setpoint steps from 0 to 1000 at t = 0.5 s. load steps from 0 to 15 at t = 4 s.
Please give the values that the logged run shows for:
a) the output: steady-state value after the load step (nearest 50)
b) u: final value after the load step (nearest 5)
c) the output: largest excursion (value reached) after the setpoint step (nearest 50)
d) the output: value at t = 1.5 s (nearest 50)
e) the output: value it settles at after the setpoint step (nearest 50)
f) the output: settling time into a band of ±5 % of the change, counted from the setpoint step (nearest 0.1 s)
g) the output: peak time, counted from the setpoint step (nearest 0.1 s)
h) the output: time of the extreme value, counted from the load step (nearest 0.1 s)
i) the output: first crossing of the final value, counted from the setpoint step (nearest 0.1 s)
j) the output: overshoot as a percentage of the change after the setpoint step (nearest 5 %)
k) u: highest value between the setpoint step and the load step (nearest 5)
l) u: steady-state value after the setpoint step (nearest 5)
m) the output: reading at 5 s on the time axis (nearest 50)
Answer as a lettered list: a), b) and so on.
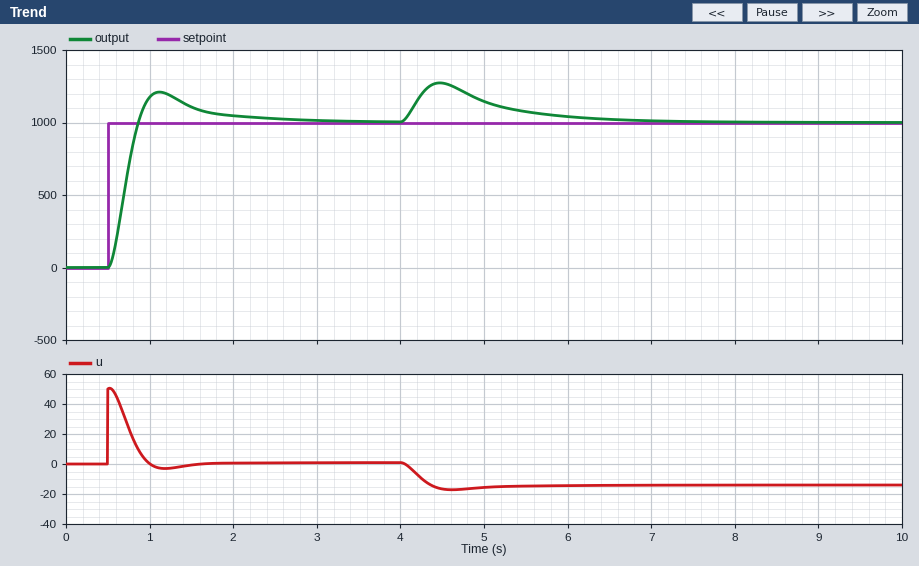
a) 1000
b) -15
c) 1200
d) 1100
e) 1000
f) 1.4 s
g) 0.6 s
h) 0.5 s
i) 0.4 s
j) 20 %
k) 50
l) 0
m) 1150
